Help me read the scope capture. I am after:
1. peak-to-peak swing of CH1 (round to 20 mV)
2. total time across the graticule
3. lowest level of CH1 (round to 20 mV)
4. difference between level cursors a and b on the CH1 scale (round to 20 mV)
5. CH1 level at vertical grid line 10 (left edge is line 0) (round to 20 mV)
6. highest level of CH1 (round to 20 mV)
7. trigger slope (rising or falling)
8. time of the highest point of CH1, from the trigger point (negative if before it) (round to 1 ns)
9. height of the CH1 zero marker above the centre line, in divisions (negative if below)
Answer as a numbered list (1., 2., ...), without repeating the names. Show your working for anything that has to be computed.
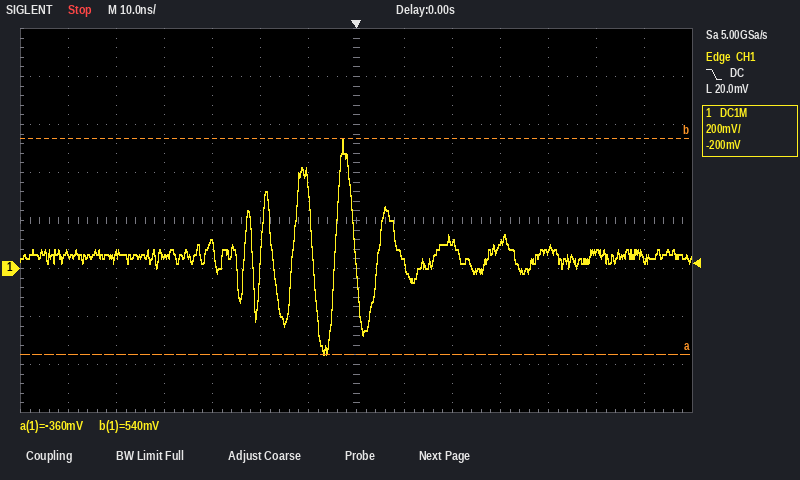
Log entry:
1. 540 mV − (-360 mV) = 900 mV
2. 140 ns
3. -360 mV
4. 900 mV
5. 100 mV
6. 540 mV
7. falling
8. -3 ns
9. -1.0 div
